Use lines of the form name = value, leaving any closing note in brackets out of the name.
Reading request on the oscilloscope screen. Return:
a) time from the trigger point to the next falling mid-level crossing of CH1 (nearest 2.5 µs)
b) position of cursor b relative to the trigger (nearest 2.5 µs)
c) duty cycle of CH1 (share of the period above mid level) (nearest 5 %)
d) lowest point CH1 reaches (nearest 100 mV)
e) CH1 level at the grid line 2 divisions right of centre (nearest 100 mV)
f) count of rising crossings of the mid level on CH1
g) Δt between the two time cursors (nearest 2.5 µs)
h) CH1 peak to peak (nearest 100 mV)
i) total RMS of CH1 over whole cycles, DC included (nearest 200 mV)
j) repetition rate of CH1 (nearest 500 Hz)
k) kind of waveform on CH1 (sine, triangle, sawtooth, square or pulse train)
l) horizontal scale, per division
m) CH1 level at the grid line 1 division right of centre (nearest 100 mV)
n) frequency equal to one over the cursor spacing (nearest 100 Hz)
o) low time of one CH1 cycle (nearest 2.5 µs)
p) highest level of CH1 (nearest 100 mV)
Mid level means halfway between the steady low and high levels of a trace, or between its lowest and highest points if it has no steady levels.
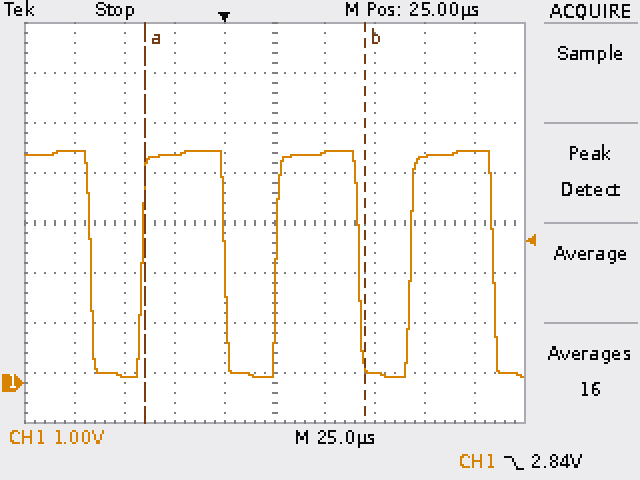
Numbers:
time from the trigger point to the next falling mid-level crossing of CH1 = 67.5 µs
position of cursor b relative to the trigger = +70.0 µs
duty cycle of CH1 (share of the period above mid level) = 60 %
lowest point CH1 reaches = 100 mV
CH1 level at the grid line 2 divisions right of centre = 200 mV
count of rising crossings of the mid level on CH1 = 3
Δt between the two time cursors = 110.0 µs
CH1 peak to peak = 4.5 V
total RMS of CH1 over whole cycles, DC included = 3.6 V
repetition rate of CH1 = 15.0 kHz
kind of waveform on CH1 = pulse train
horizontal scale, per division = 25 µs
CH1 level at the grid line 1 division right of centre = 4.6 V
frequency equal to one over the cursor spacing = 9.1 kHz
low time of one CH1 cycle = 25.0 µs
highest level of CH1 = 4.6 V
